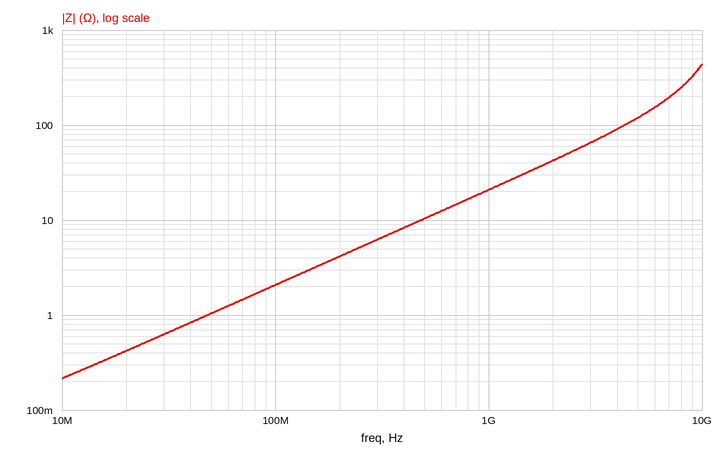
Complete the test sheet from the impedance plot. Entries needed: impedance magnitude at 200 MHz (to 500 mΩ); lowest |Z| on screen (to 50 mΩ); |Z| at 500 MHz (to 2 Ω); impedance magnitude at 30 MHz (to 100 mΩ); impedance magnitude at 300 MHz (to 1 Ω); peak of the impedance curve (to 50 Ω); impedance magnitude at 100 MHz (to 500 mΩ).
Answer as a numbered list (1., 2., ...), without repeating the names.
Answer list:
1. 4.0 Ω
2. 200 mΩ
3. 10 Ω
4. 600 mΩ
5. 6 Ω
6. 450 Ω
7. 2.0 Ω
